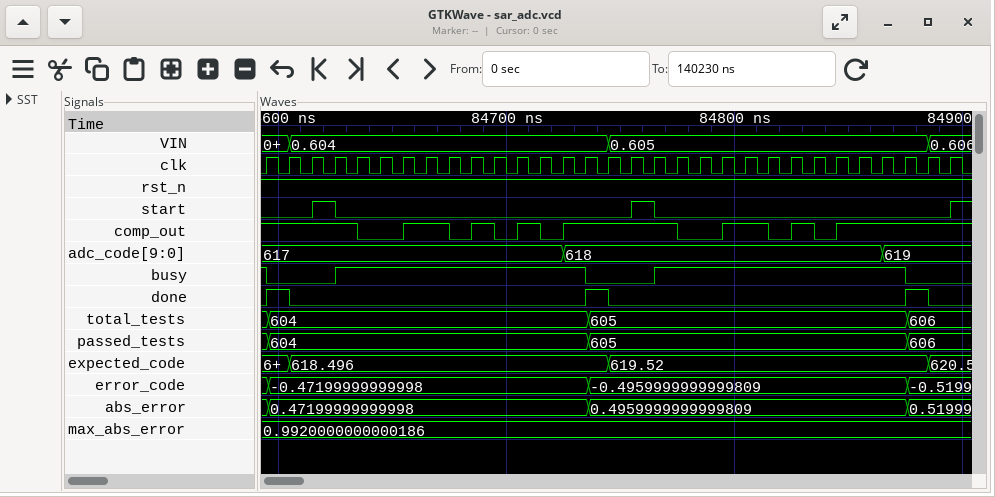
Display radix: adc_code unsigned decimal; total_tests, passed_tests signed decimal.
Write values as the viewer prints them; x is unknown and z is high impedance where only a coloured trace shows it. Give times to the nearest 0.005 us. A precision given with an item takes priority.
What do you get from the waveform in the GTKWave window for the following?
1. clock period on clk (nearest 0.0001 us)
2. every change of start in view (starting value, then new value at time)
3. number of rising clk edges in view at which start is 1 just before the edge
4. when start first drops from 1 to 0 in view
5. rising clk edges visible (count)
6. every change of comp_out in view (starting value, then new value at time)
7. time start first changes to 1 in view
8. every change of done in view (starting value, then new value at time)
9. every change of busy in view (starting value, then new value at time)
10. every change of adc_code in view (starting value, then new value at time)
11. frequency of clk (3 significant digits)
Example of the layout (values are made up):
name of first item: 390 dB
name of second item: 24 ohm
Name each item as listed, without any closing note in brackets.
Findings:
clock period on clk: 0.01 us
every change of start in view: 0, 1 at 84.615 us, 0 at 84.625 us, 1 at 84.755 us, 0 at 84.765 us, 1 at 84.895 us
number of rising clk edges in view at which start is 1 just before the edge: 2
when start first drops from 1 to 0 in view: 84.625 us
rising clk edges visible: 31
every change of comp_out in view: 1, 0 at 84.635 us, 1 at 84.655 us, 0 at 84.675 us, 1 at 84.685 us, 0 at 84.695 us, 1 at 84.705 us, 0 at 84.715 us, 1 at 84.725 us, 0 at 84.775 us, 1 at 84.795 us, 0 at 84.815 us, 1 at 84.825 us, 0 at 84.835 us, 1 at 84.845 us
time start first changes to 1 in view: 84.615 us
every change of done in view: 0, 1 at 84.595 us, 0 at 84.605 us, 1 at 84.735 us, 0 at 84.745 us, 1 at 84.875 us, 0 at 84.885 us
every change of busy in view: 1, 0 at 84.595 us, 1 at 84.625 us, 0 at 84.735 us, 1 at 84.765 us, 0 at 84.875 us
every change of adc_code in view: 617, 618 at 84.725 us, 619 at 84.865 us
frequency of clk: 100 MHz
